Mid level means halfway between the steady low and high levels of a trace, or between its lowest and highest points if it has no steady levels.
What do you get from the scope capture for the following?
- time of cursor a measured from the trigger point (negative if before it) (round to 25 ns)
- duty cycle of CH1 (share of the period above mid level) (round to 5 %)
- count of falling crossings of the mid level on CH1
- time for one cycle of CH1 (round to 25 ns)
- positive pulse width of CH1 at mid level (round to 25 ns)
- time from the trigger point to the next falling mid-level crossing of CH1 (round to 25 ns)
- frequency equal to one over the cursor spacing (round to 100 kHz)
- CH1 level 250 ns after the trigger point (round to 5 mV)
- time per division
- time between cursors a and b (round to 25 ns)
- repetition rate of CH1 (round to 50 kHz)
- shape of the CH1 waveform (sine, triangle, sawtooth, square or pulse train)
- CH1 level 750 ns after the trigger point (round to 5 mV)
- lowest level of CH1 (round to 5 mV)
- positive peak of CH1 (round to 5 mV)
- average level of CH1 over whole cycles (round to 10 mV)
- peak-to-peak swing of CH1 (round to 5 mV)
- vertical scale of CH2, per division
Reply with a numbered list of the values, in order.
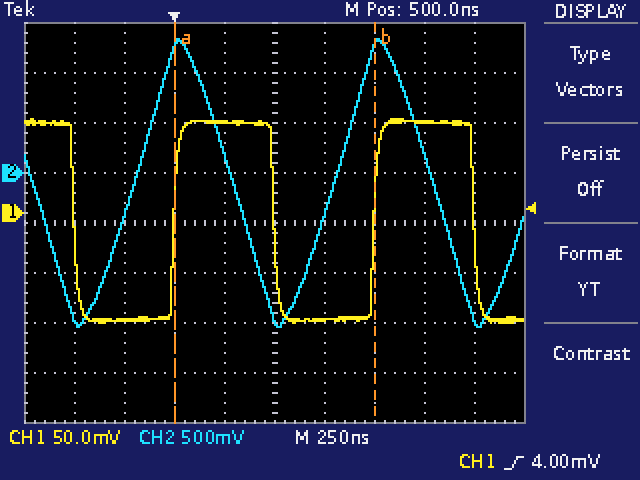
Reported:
1. 0 ns
2. 50 %
3. 3
4. 1.000 µs
5. 500 ns
6. 500 ns
7. 1.0 MHz
8. 90 mV
9. 250 ns
10. 1.000 µs
11. 1.00 MHz
12. square
13. -105 mV
14. -110 mV
15. 95 mV
16. -10 mV
17. 205 mV
18. 500 mV
